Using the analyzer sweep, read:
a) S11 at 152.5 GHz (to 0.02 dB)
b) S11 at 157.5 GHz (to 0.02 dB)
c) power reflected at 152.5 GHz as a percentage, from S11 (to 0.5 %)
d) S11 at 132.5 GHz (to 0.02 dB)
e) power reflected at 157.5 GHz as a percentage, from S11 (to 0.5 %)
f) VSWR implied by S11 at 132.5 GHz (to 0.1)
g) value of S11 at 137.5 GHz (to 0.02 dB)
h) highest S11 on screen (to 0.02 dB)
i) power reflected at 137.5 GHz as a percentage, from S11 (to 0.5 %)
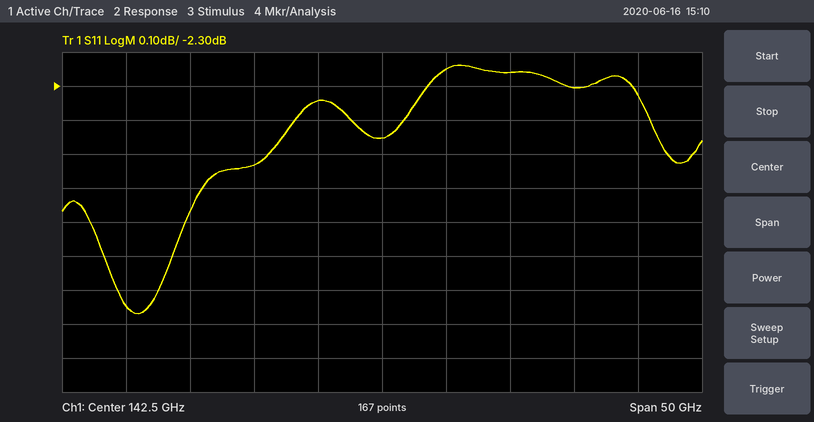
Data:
-2.26 dB
-2.30 dB
59.5 %
-2.54 dB
59.0 %
6.9
-2.34 dB
-2.24 dB
58.5 %
